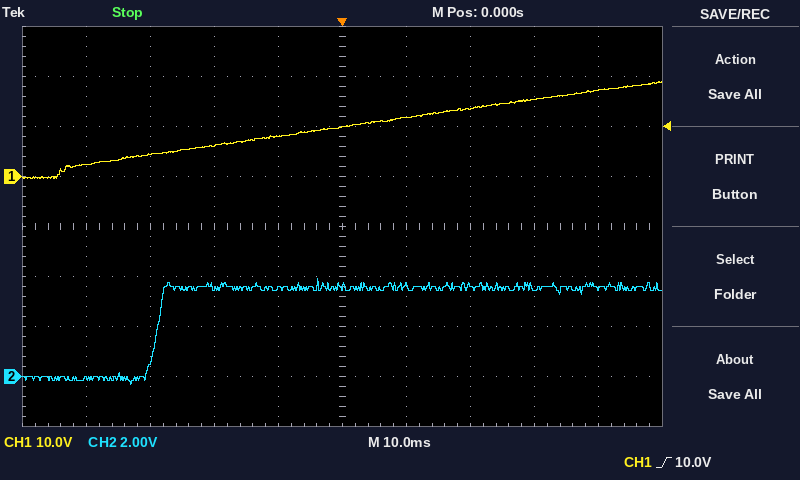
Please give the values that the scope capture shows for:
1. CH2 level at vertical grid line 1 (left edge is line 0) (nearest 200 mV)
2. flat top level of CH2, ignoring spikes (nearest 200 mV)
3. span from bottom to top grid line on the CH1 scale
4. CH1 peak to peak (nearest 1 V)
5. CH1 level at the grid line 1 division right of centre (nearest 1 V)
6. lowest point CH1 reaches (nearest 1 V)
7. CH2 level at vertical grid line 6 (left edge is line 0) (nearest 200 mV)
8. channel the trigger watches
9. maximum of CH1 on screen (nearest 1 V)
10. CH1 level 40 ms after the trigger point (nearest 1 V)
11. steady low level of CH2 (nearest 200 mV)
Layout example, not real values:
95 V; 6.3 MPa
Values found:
0.0 V; 3.6 V; 80 V; 19 V; 12 V; 0 V; 3.6 V; CH1; 19 V; 17 V; 0.0 V
